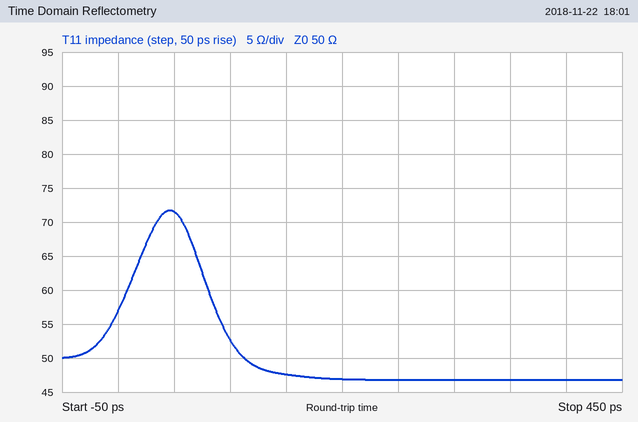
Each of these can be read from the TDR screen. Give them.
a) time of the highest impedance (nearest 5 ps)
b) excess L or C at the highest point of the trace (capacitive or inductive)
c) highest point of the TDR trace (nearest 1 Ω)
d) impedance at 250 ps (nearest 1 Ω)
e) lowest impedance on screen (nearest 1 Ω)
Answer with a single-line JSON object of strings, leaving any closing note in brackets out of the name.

{"time of the highest impedance": "45 ps", "excess L or C at the highest point of the trace": "inductive", "highest point of the TDR trace": "72 Ω", "impedance at 250 ps": "47 Ω", "lowest impedance on screen": "47 Ω"}
